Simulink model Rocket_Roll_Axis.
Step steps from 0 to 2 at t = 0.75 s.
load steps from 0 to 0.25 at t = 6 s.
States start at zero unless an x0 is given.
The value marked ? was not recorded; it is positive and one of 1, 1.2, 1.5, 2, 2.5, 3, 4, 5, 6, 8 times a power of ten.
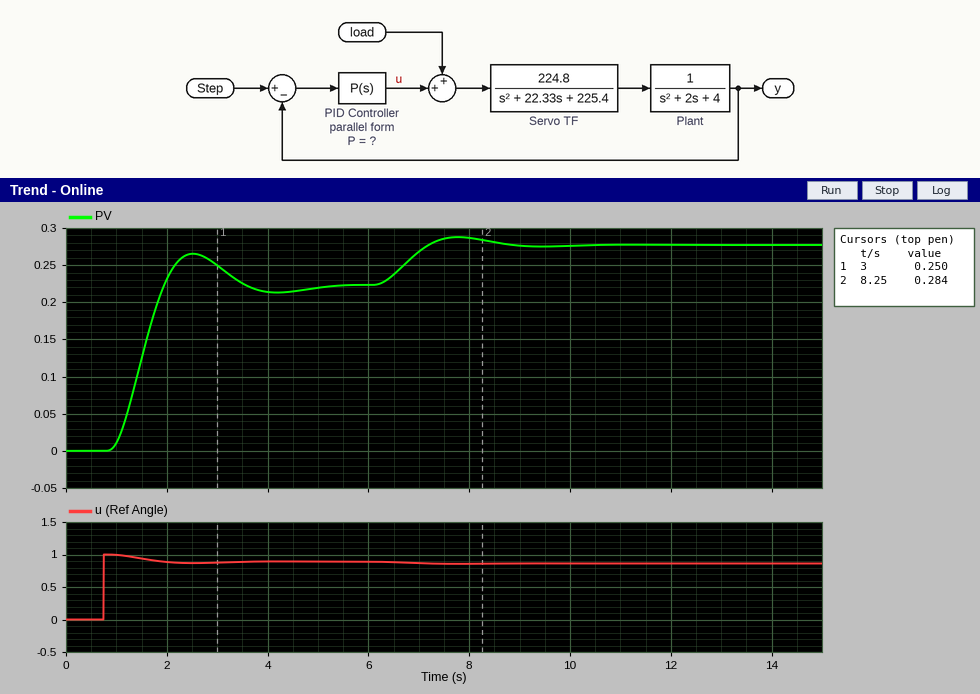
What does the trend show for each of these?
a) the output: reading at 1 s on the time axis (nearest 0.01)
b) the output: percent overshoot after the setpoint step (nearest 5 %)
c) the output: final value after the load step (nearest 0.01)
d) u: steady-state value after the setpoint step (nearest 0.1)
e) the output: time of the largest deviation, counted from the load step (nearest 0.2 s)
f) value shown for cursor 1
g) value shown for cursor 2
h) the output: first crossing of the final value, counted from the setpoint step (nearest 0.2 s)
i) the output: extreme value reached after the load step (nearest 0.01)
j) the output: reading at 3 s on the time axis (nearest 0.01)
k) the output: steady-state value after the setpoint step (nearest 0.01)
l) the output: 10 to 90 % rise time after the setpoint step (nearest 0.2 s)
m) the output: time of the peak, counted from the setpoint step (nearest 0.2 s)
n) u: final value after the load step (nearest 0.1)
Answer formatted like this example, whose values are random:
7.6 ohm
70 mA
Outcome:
0.01
20 %
0.28
0.9
1.8 s
0.250
0.284
1.2 s
0.29
0.25
0.22
0.8 s
1.8 s
0.9
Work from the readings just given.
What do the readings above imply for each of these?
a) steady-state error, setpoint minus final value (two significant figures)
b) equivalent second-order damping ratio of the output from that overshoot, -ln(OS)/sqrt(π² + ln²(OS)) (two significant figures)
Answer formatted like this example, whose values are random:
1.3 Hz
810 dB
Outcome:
1.8
0.46
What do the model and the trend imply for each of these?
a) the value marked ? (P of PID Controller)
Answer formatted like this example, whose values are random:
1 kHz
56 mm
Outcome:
0.5
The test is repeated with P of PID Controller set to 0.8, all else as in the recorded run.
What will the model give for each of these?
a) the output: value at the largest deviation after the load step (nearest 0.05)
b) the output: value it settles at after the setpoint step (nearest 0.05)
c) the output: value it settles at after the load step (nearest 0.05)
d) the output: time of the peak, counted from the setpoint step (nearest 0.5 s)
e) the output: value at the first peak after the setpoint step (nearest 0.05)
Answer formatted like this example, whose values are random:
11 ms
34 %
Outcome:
0.40
0.35
0.40
1.5 s
0.40
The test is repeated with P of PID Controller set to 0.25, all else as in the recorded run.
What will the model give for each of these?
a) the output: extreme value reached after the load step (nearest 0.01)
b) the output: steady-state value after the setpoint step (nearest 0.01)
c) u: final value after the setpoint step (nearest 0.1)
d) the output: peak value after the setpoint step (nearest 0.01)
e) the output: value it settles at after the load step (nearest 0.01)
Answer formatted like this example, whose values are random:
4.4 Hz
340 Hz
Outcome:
0.19
0.12
0.5
0.14
0.18
